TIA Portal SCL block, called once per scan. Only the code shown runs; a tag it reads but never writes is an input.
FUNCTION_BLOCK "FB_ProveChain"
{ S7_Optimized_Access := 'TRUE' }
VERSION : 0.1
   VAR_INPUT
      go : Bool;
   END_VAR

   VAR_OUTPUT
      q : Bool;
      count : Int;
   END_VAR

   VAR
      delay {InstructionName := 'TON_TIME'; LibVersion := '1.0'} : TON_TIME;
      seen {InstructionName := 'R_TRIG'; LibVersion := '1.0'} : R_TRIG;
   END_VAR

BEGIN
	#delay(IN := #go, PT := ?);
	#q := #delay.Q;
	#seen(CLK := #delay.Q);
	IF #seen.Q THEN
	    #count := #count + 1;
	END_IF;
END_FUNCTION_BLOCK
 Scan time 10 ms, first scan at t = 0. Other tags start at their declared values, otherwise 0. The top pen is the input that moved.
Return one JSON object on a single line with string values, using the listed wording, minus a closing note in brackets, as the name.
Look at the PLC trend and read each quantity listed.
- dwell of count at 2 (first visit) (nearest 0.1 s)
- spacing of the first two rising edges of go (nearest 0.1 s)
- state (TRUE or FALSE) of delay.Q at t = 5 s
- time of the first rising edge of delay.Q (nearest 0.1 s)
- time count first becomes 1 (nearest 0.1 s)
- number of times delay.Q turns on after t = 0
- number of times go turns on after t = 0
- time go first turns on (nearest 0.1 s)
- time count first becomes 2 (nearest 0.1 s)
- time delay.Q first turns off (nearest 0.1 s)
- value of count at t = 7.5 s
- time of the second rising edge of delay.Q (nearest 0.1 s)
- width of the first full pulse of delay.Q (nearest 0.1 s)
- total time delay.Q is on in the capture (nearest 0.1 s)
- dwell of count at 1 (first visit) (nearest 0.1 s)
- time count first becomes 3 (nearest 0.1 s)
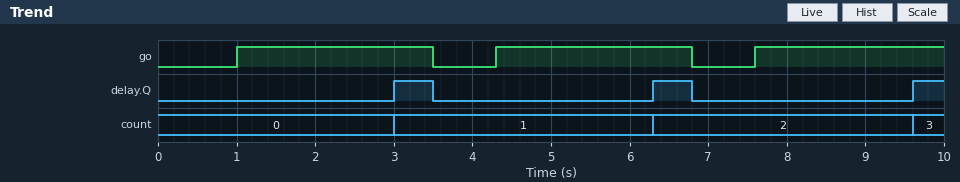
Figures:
{"dwell of count at 2 (first visit)": "3.3 s", "spacing of the first two rising edges of go": "3.3 s", "state (TRUE or FALSE) of delay.Q at t = 5 s": "FALSE", "time of the first rising edge of delay.Q": "3.0 s", "time count first becomes 1": "3.0 s", "number of times delay.Q turns on after t = 0": "3", "number of times go turns on after t = 0": "3", "time go first turns on": "1.0 s", "time count first becomes 2": "6.3 s", "time delay.Q first turns off": "3.5 s", "value of count at t = 7.5 s": "2", "time of the second rising edge of delay.Q": "6.3 s", "width of the first full pulse of delay.Q": "0.5 s", "total time delay.Q is on in the capture": "1.4 s", "dwell of count at 1 (first visit)": "3.3 s", "time count first becomes 3": "9.6 s"}
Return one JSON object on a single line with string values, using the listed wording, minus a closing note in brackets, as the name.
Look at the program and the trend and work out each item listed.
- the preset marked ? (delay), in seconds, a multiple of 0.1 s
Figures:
{"the preset marked ? (delay), in seconds, a multiple of 0.1 s": "2.0 s"}
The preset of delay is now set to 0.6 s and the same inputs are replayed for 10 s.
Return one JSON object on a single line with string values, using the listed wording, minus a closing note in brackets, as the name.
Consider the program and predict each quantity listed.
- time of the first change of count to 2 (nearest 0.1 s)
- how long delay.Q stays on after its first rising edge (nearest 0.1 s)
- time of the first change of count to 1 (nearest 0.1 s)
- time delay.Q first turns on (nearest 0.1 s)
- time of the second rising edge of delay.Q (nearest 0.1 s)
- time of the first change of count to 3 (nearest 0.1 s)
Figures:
{"time of the first change of count to 2": "4.9 s", "how long delay.Q stays on after its first rising edge": "1.9 s", "time of the first change of count to 1": "1.6 s", "time delay.Q first turns on": "1.6 s", "time of the second rising edge of delay.Q": "4.9 s", "time of the first change of count to 3": "8.2 s"}
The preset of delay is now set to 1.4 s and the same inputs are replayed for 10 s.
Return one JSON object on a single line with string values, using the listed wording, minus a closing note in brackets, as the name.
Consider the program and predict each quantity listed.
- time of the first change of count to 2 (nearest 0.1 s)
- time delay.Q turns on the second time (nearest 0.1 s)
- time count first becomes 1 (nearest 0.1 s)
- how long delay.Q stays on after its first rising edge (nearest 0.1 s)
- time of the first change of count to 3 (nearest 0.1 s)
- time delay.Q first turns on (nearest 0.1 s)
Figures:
{"time of the first change of count to 2": "5.7 s", "time delay.Q turns on the second time": "5.7 s", "time count first becomes 1": "2.4 s", "how long delay.Q stays on after its first rising edge": "1.1 s", "time of the first change of count to 3": "9.0 s", "time delay.Q first turns on": "2.4 s"}
